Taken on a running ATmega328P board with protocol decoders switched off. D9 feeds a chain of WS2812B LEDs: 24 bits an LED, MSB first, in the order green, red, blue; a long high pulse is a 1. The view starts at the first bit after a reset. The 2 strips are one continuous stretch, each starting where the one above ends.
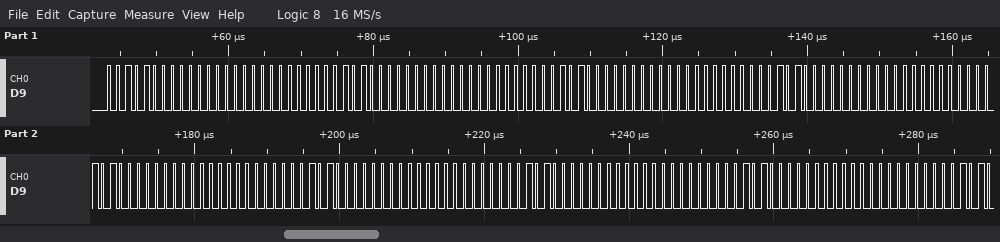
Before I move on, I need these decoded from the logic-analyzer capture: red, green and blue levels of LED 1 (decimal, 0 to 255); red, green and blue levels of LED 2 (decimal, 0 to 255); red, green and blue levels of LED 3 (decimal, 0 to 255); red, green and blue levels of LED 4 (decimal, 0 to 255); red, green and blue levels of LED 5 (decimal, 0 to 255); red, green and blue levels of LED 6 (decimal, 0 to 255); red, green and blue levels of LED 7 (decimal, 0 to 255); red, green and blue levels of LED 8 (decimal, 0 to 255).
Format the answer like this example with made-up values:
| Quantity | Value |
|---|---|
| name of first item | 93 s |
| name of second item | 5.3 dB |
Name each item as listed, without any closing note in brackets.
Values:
| Quantity | Value |
|---|---|
| red, green and blue levels of LED 1 | 0, 40, 0 |
| red, green and blue levels of LED 2 | 0, 40, 0 |
| red, green and blue levels of LED 3 | 0, 40, 0 |
| red, green and blue levels of LED 4 | 0, 40, 0 |
| red, green and blue levels of LED 5 | 0, 40, 0 |
| red, green and blue levels of LED 6 | 0, 40, 0 |
| red, green and blue levels of LED 7 | 0, 40, 0 |
| red, green and blue levels of LED 8 | 0, 40, 0 |
